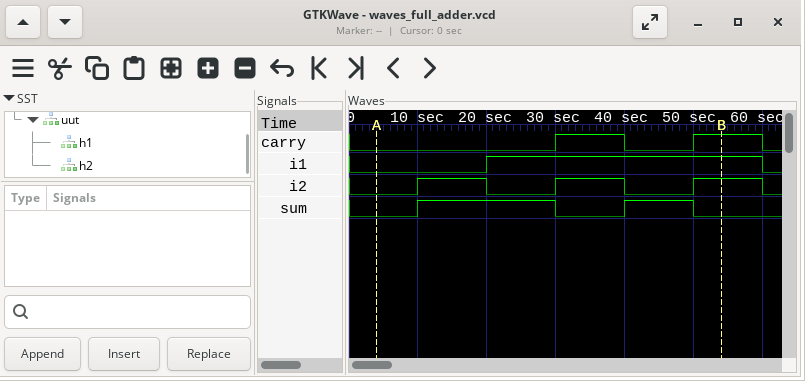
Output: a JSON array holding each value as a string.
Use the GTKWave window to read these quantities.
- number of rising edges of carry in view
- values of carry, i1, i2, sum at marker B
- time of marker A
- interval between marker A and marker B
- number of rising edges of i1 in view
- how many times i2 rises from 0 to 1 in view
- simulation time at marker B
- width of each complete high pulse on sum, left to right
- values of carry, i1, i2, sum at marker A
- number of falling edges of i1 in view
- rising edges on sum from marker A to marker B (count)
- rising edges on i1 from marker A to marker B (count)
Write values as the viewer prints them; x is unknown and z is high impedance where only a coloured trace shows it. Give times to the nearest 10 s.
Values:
["2", "carry=1, i1=1, i2=1, sum=0", "0 s", "50 s", "1", "3", "50 s", "20 s, 10 s", "carry=0, i1=0, i2=0, sum=0", "1", "2", "1"]
